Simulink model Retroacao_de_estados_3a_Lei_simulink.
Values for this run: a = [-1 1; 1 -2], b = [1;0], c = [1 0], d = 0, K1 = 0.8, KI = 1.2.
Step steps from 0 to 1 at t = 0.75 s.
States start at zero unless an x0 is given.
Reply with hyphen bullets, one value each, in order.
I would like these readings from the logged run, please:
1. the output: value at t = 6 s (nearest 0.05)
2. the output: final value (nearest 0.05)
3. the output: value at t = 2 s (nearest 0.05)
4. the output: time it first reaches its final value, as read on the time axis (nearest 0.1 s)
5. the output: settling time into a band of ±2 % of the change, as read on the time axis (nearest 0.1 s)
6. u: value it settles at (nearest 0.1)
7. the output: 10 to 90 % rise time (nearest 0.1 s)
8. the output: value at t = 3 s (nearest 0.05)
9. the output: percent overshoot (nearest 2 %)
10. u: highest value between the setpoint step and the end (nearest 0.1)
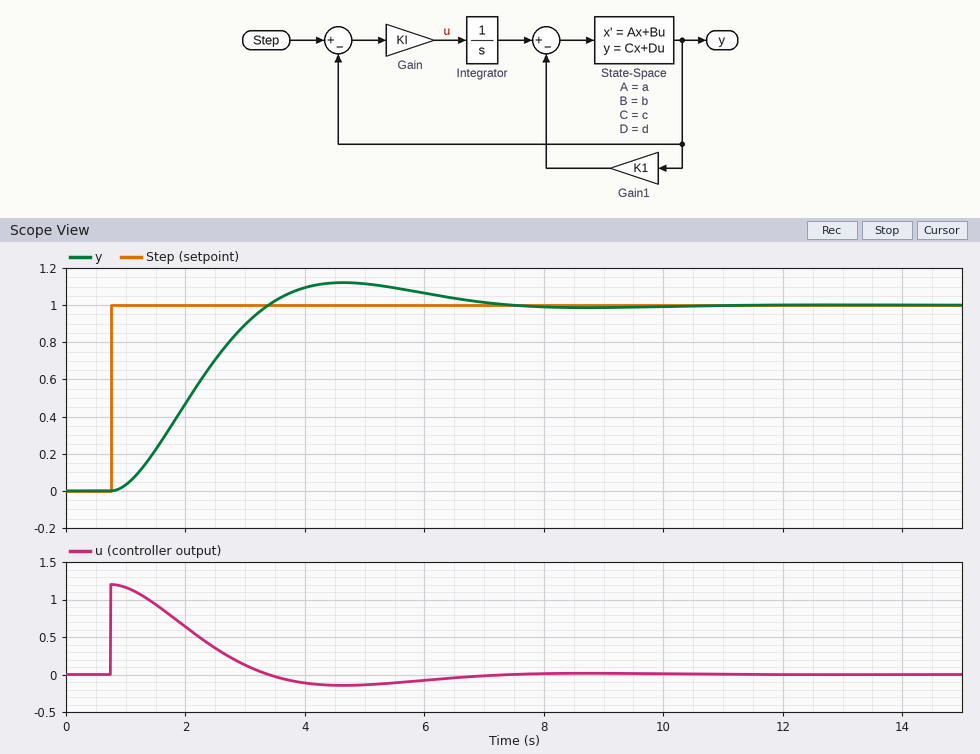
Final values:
- 1.05
- 1.00
- 0.45
- 3.4 s
- 6.9 s
- 0.0
- 1.8 s
- 0.90
- 12 %
- 1.2
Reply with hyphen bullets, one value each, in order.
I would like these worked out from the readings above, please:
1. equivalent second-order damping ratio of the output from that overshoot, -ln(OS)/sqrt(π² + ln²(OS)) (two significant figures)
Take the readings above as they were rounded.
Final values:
- 0.56
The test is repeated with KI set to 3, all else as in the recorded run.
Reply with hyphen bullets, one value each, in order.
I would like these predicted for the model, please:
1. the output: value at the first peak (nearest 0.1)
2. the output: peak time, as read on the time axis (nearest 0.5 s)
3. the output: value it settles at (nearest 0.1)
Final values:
- 1.3
- 3.0 s
- 1.0
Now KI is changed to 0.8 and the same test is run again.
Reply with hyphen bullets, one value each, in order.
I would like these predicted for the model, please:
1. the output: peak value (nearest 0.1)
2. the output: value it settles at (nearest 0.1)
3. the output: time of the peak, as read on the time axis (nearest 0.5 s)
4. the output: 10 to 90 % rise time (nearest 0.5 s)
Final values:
- 1.1
- 1.0
- 6.0 s
- 2.5 s
